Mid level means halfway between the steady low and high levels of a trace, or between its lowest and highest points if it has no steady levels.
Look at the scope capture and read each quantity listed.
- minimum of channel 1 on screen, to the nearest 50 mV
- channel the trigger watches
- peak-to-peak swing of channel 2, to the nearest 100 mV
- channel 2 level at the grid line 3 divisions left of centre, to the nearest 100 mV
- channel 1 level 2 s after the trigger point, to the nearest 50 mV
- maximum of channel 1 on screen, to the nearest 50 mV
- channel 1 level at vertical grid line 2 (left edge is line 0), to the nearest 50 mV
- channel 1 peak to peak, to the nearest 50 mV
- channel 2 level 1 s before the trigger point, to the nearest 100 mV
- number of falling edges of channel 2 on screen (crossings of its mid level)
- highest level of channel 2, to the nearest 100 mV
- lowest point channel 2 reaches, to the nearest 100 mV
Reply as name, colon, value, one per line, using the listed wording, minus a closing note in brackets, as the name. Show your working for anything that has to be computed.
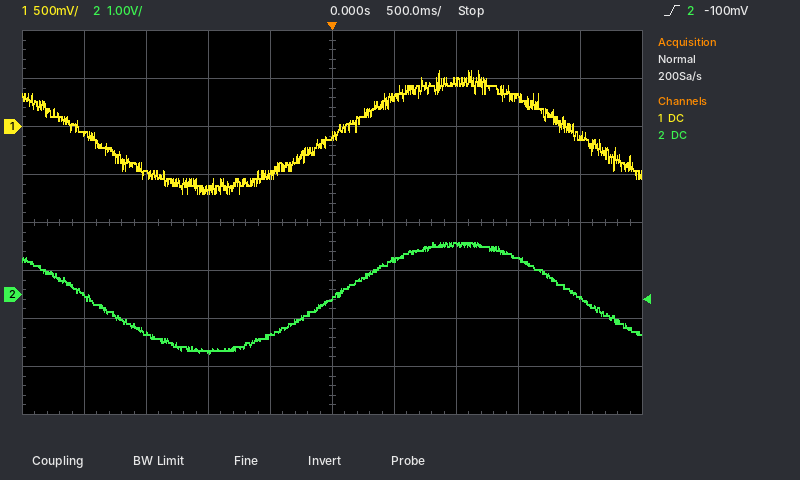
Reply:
minimum of channel 1 on screen, to the nearest 50 mV: -700 mV
channel the trigger watches: channel 2
peak-to-peak swing of channel 2, to the nearest 100 mV: 1.1 V − (-1.2 V) = 2.3 V
channel 2 level at the grid line 3 divisions left of centre, to the nearest 100 mV: -800 mV
channel 1 level 2 s after the trigger point, to the nearest 50 mV: -100 mV
maximum of channel 1 on screen, to the nearest 50 mV: 600 mV
channel 1 level at vertical grid line 2 (left edge is line 0), to the nearest 50 mV: -500 mV
channel 1 peak to peak, to the nearest 50 mV: 600 mV − (-700 mV) = 1.30 V
channel 2 level 1 s before the trigger point, to the nearest 100 mV: -1.2 V
number of falling edges of channel 2 on screen: 2
highest level of channel 2, to the nearest 100 mV: 1.1 V
lowest point channel 2 reaches, to the nearest 100 mV: -1.2 V
